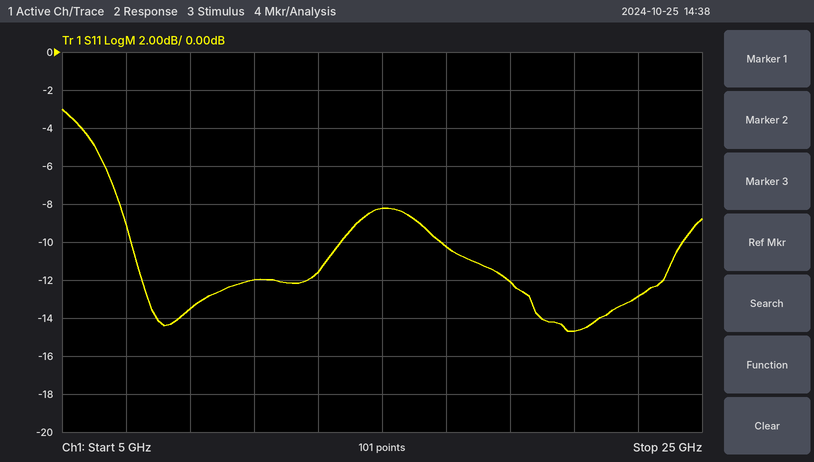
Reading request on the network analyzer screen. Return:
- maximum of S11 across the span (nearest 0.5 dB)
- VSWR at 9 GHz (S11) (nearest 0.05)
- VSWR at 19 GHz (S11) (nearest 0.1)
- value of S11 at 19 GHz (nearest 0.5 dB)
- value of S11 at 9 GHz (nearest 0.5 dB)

-3.0 dB
1.55
1.7
-12.0 dB
-13.5 dB
